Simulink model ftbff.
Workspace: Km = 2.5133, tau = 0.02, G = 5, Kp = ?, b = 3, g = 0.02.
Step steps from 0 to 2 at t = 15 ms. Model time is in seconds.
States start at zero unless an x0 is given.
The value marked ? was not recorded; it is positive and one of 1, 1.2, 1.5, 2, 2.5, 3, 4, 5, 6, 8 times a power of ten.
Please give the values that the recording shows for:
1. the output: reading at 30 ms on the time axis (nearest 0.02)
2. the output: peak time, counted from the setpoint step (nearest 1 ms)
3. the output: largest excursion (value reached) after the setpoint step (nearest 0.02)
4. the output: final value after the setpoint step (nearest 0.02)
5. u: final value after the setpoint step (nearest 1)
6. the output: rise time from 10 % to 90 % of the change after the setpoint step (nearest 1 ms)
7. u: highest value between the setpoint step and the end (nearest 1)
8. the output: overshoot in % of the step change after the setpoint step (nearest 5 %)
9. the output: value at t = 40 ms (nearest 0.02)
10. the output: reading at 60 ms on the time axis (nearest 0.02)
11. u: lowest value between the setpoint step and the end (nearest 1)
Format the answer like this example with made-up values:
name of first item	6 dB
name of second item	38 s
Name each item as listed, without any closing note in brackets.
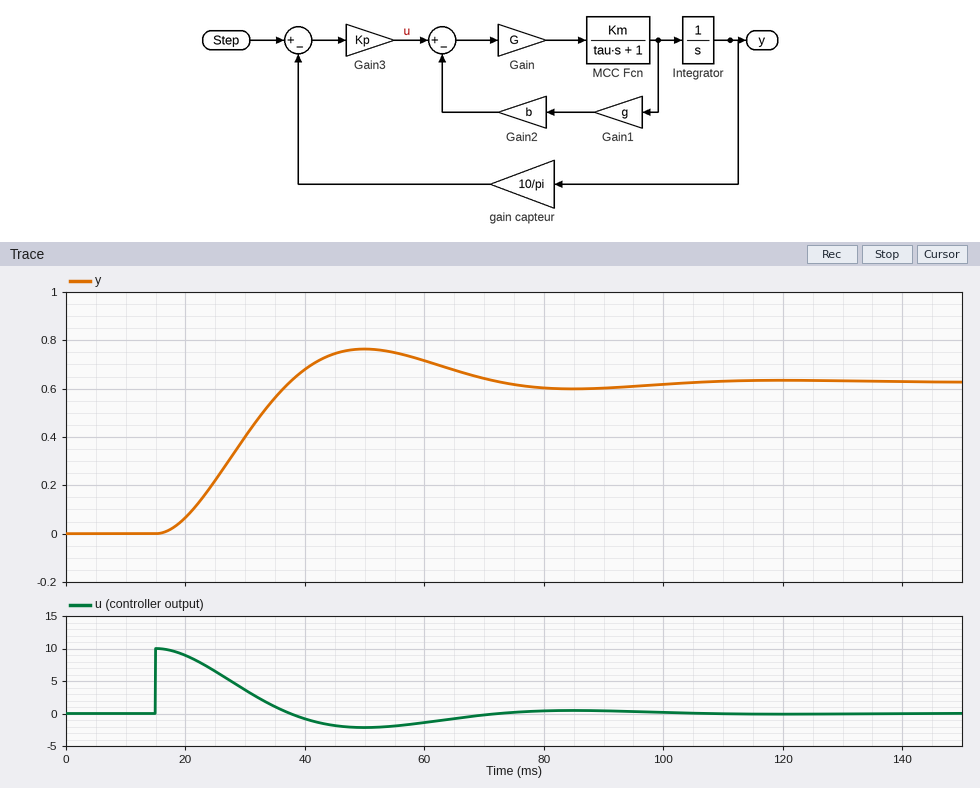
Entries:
the output: reading at 30 ms on the time axis	0.40
the output: peak time, counted from the setpoint step	35 ms
the output: largest excursion (value reached) after the setpoint step	0.76
the output: final value after the setpoint step	0.62
u: final value after the setpoint step	0
the output: rise time from 10 % to 90 % of the change after the setpoint step	15 ms
u: highest value between the setpoint step and the end	10
the output: overshoot in % of the step change after the setpoint step	20 %
the output: value at t = 40 ms	0.68
the output: reading at 60 ms on the time axis	0.72
u: lowest value between the setpoint step and the end	-2
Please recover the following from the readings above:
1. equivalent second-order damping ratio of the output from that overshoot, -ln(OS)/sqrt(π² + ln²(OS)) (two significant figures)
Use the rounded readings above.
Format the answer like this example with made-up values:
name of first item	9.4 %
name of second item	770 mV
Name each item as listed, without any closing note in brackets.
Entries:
equivalent second-order damping ratio of the output from that overshoot, -ln(OS)/sqrt(π² + ln²(OS))	0.46
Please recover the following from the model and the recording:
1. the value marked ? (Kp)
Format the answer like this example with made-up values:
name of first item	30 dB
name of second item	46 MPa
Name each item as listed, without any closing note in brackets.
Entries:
the value marked ?	5
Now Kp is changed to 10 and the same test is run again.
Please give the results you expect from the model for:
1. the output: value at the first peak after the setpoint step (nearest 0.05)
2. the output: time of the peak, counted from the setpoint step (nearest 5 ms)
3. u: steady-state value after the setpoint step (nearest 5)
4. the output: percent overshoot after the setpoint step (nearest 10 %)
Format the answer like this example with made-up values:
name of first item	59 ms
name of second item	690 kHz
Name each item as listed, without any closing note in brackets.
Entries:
the output: value at the first peak after the setpoint step	0.85
the output: time of the peak, counted from the setpoint step	25 ms
u: steady-state value after the setpoint step	0
the output: percent overshoot after the setpoint step	40 %
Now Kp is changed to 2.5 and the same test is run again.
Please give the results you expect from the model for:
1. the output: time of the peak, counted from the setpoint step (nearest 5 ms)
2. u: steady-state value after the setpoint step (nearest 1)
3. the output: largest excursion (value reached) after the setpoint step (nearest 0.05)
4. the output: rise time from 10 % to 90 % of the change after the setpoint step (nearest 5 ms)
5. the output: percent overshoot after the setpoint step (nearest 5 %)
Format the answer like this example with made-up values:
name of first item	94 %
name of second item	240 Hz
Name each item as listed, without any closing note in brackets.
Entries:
the output: time of the peak, counted from the setpoint step	55 ms
u: steady-state value after the setpoint step	0
the output: largest excursion (value reached) after the setpoint step	0.70
the output: rise time from 10 % to 90 % of the change after the setpoint step	25 ms
the output: percent overshoot after the setpoint step	10 %
